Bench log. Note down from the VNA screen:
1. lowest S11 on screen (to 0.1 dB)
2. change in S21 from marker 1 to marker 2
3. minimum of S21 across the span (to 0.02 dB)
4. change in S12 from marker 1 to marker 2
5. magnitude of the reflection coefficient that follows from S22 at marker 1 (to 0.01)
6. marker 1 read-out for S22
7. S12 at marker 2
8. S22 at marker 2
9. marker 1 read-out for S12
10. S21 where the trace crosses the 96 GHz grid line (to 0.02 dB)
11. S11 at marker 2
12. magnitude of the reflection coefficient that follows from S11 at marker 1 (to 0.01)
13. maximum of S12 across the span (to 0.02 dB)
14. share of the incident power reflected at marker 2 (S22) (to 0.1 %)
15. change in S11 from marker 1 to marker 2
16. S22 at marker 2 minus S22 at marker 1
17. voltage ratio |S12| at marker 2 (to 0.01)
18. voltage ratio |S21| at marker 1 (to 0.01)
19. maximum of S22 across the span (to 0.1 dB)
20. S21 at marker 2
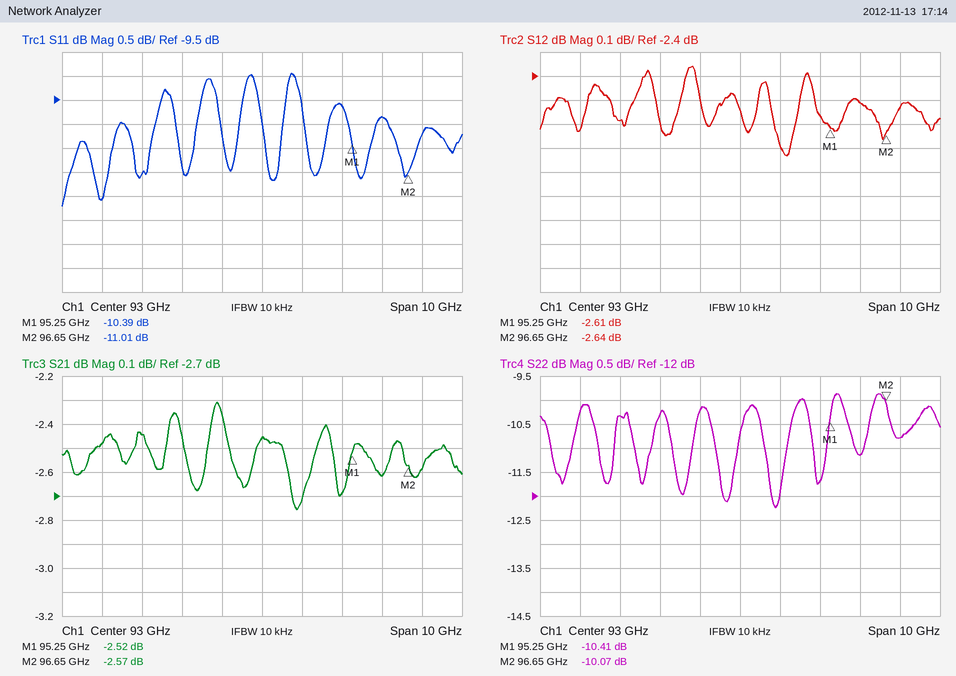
-11.7 dB
-0.05 dB
-2.76 dB
-0.03 dB
0.30
-10.41 dB
-2.64 dB
-10.07 dB
-2.61 dB
-2.62 dB
-11.01 dB
0.30
-2.36 dB
9.8 %
-0.62 dB
0.34 dB
0.74
0.75
-9.9 dB
-2.57 dB
